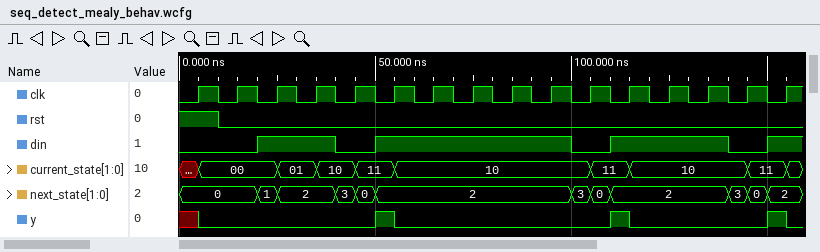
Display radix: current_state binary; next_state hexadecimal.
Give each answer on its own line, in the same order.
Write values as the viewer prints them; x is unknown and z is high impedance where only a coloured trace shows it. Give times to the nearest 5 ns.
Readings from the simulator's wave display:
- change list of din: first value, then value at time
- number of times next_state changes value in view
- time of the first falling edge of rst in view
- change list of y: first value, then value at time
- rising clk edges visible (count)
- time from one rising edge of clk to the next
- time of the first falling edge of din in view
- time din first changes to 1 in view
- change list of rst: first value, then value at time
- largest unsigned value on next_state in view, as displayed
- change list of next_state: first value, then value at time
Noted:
0, 1 at 20 ns, 0 at 40 ns, 1 at 50 ns, 0 at 100 ns, 1 at 110 ns, 0 at 140 ns, 1 at 150 ns
11
10 ns
x, 0 at 5 ns, 1 at 50 ns, 0 at 55 ns, 1 at 110 ns, 0 at 115 ns, 1 at 150 ns, 0 at 155 ns
16
10 ns
40 ns
20 ns
1, 0 at 10 ns
3
0, 1 at 20 ns, 2 at 25 ns, 3 at 40 ns, 0 at 45 ns, 2 at 50 ns, 3 at 100 ns, 0 at 105 ns, 2 at 110 ns, 3 at 140 ns, 0 at 145 ns, 2 at 150 ns
